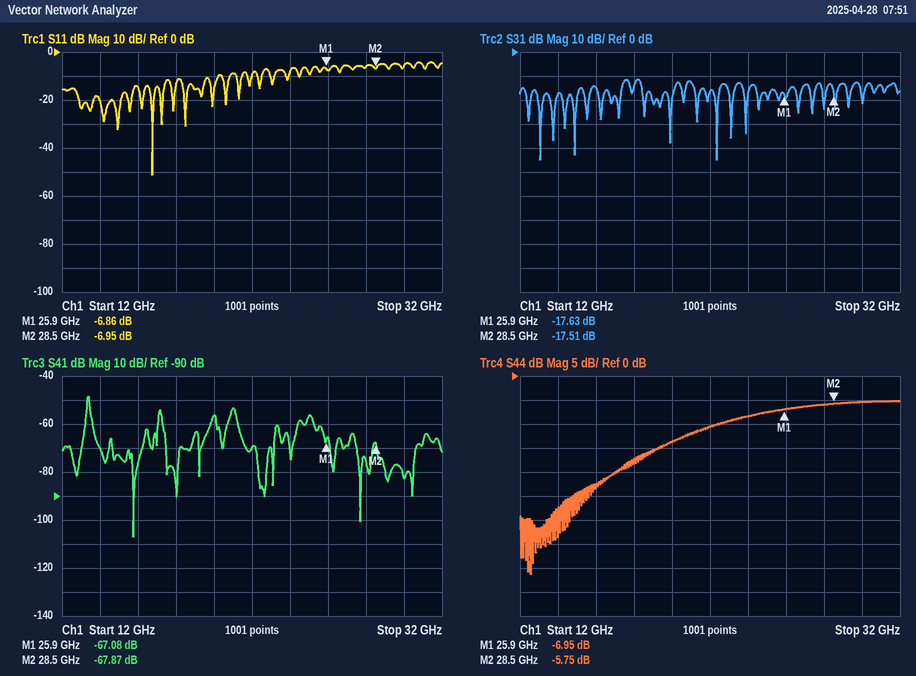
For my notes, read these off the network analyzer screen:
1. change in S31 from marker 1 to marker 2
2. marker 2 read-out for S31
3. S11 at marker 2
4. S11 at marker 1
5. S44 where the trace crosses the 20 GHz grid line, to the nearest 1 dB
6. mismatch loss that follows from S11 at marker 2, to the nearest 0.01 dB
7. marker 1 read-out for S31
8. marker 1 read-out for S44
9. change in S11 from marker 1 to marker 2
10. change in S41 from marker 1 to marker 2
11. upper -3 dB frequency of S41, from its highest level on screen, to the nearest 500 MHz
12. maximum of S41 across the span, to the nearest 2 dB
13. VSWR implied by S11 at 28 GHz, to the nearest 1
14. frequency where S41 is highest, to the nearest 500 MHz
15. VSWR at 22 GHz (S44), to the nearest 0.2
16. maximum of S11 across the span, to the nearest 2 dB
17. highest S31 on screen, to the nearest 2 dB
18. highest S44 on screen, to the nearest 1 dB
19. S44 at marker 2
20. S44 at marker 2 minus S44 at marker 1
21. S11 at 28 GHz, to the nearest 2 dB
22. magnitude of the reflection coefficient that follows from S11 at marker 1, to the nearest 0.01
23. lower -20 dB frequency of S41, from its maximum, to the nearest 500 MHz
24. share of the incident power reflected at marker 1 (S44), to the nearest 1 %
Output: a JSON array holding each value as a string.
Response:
["0.12 dB", "-17.51 dB", "-6.95 dB", "-6.86 dB", "-14 dB", "0.98 dB", "-17.63 dB", "-6.95 dB", "-0.09 dB", "-0.79 dB", "13.5 GHz", "-48 dB", "3", "13.5 GHz", "1.8", "-4 dB", "-12 dB", "-5 dB", "-5.75 dB", "1.20 dB", "-6 dB", "0.45", "13.0 GHz", "20 %"]
